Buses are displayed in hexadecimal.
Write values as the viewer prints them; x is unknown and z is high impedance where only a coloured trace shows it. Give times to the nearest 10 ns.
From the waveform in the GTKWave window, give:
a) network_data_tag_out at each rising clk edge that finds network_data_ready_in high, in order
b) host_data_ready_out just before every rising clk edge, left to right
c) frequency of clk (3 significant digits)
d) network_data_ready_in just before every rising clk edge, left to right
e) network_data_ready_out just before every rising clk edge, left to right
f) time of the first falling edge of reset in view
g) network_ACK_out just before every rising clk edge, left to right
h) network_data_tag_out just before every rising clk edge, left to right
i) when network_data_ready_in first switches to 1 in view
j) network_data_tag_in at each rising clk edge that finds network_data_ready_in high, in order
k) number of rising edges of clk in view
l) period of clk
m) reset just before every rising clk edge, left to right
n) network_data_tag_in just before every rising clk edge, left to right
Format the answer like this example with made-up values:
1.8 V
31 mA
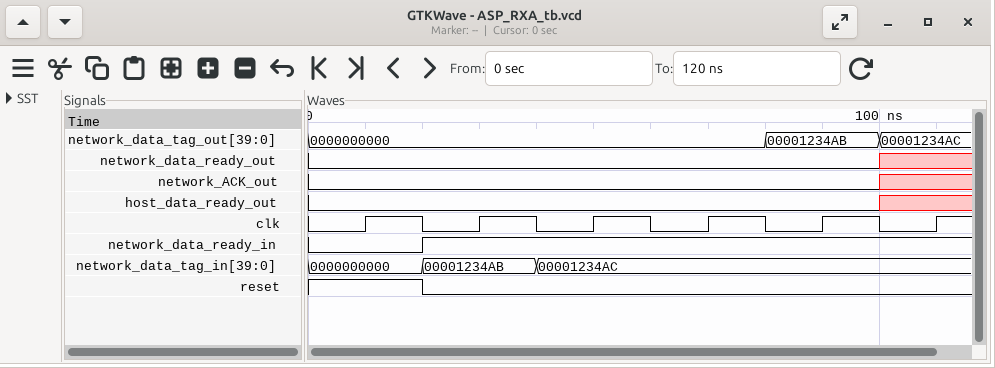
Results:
0000000000, 0000000000, 0000000000, 00001234AB, 00001234AC
0 0 0 0 0 x
50.0 MHz
0 1 1 1 1 1
0 0 0 0 0 x
20 ns
0 0 0 0 0 x
0000000000, 0000000000, 0000000000, 0000000000, 00001234AB, 00001234AC
20 ns
00001234AB, 00001234AC, 00001234AC, 00001234AC, 00001234AC
6
20 ns
1 0 0 0 0 0
0000000000, 00001234AB, 00001234AC, 00001234AC, 00001234AC, 00001234AC
